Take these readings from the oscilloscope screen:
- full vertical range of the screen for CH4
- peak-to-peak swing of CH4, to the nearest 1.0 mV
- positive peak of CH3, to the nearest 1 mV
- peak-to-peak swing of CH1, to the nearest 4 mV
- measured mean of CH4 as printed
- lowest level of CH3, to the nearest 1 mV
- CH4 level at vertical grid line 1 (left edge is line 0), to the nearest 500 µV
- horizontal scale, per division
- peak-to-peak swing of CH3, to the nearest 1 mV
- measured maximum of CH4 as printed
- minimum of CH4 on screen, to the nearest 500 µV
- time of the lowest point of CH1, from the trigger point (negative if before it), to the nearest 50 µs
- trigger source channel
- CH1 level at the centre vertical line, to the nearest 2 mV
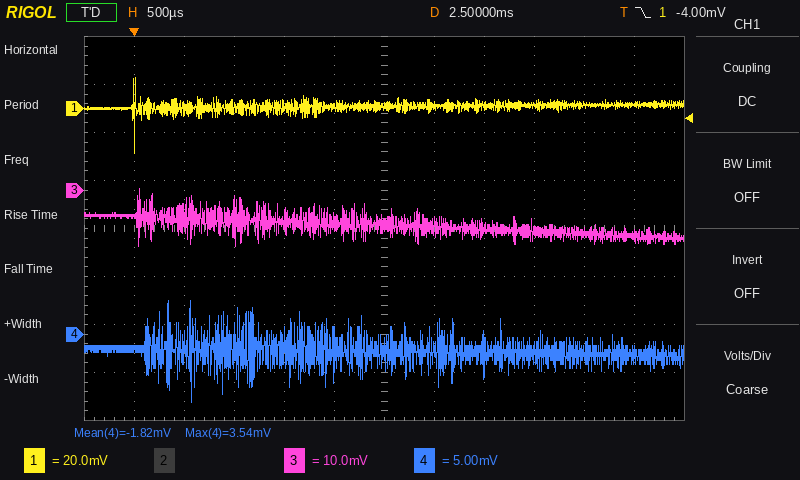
40 mV
11.0 mV
0 mV
32 mV
-1.82 mV
-12 mV
-1.5 mV
500 µs
12 mV
3.54 mV
-7.0 mV
0 µs
CH1
0 mV
